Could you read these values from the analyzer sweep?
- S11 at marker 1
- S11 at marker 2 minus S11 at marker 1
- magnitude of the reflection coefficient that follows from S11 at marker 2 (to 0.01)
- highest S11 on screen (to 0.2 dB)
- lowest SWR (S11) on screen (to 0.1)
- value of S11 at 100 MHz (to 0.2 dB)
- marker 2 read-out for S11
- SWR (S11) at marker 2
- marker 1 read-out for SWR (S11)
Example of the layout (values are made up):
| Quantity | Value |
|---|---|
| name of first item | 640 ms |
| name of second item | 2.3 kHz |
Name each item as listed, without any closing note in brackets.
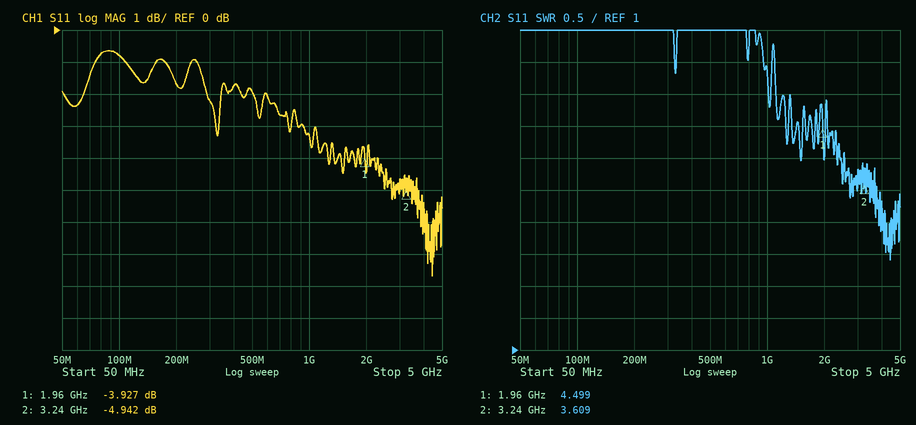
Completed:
| Quantity | Value |
|---|---|
| S11 at marker 1 | -3.927 dB |
| S11 at marker 2 minus S11 at marker 1 | -1.015 dB |
| magnitude of the reflection coefficient that follows from S11 at marker 2 | 0.57 |
| highest S11 on screen | -0.6 dB |
| lowest SWR (S11) on screen | 2.4 |
| value of S11 at 100 MHz | -0.8 dB |
| marker 2 read-out for S11 | -4.942 dB |
| SWR (S11) at marker 2 | 3.609 |
| marker 1 read-out for SWR | 4.499 |
